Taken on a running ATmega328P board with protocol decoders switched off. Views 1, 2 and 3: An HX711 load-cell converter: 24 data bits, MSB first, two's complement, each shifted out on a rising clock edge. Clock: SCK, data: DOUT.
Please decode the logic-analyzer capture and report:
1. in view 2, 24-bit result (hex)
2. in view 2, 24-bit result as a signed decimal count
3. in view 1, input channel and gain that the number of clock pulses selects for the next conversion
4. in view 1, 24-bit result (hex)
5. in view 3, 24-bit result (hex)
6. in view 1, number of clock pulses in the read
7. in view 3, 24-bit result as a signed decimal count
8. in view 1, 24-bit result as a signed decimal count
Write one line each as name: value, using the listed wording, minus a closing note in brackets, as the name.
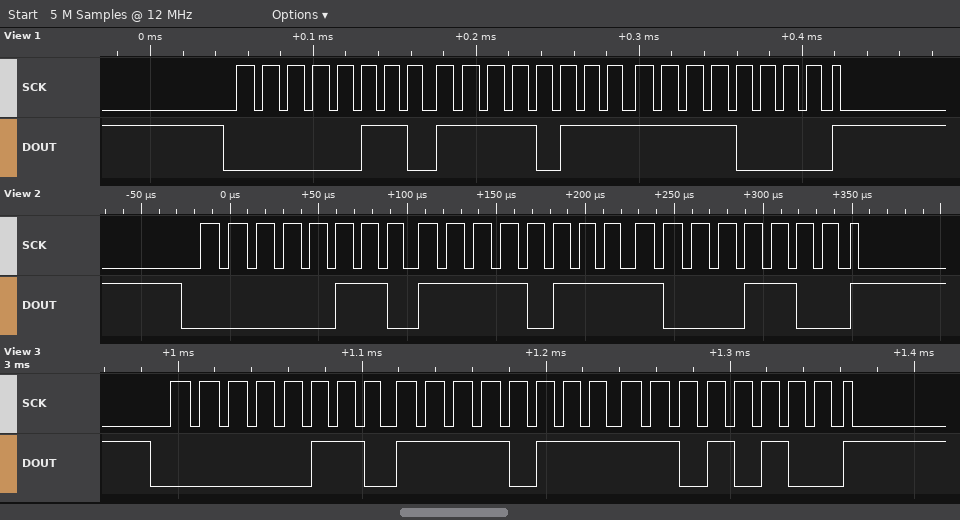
in view 2, 24-bit result: 0x06F78C
in view 2, 24-bit result as a signed decimal count: 456588
in view 1, input channel and gain that the number of clock pulses selects for the next conversion: channel A, gain 128
in view 1, 24-bit result: 0x06F7F0
in view 3, 24-bit result: 0x06F7D4
in view 1, number of clock pulses in the read: 25
in view 3, 24-bit result as a signed decimal count: 456660
in view 1, 24-bit result as a signed decimal count: 456688
